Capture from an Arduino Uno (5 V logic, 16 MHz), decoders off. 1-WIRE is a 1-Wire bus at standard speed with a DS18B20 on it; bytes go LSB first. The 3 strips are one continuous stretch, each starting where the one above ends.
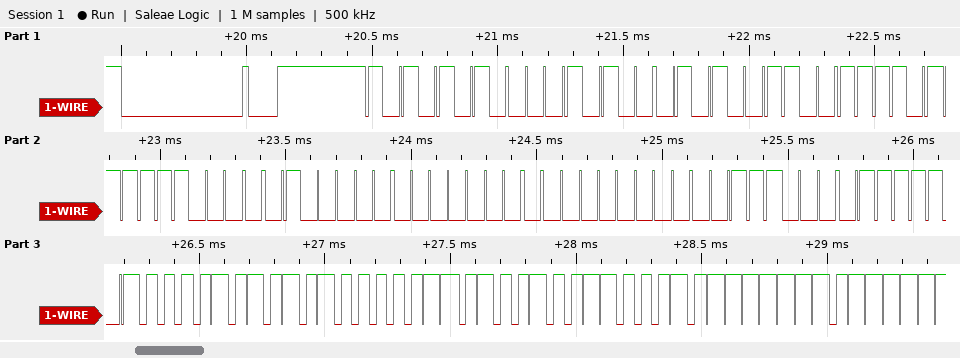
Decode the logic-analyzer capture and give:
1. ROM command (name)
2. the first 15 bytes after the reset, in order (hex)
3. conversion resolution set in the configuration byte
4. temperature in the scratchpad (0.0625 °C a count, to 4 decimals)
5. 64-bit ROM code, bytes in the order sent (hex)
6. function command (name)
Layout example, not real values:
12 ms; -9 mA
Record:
Match ROM; 55 28 CA BC 1F 04 00 00 1C BE 50 05 4B 46 7F; 12 bits; 85.0000 °C; 28 CA BC 1F 04 00 00 1C; Read Scratchpad
